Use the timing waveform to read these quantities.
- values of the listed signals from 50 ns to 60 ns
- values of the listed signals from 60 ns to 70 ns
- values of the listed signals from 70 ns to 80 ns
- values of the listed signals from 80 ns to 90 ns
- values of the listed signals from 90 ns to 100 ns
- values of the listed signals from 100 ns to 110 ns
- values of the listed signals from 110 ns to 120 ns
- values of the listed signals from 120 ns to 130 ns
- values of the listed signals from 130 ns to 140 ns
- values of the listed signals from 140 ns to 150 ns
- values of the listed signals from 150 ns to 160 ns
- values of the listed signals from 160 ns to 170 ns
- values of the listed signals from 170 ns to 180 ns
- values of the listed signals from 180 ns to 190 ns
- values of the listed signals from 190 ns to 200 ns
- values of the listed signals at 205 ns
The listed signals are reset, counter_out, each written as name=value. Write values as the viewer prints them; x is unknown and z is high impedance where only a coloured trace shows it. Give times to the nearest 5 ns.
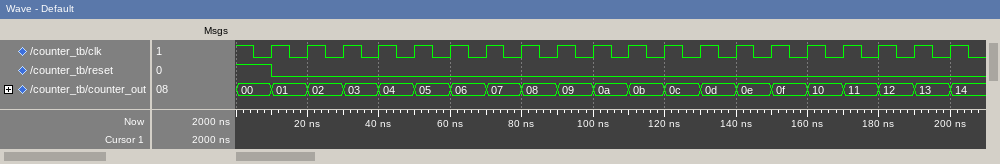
reset=0, counter_out=05
reset=0, counter_out=06
reset=0, counter_out=07
reset=0, counter_out=08
reset=0, counter_out=09
reset=0, counter_out=0a
reset=0, counter_out=0b
reset=0, counter_out=0c
reset=0, counter_out=0d
reset=0, counter_out=0e
reset=0, counter_out=0f
reset=0, counter_out=10
reset=0, counter_out=11
reset=0, counter_out=12
reset=0, counter_out=13
reset=0, counter_out=14
